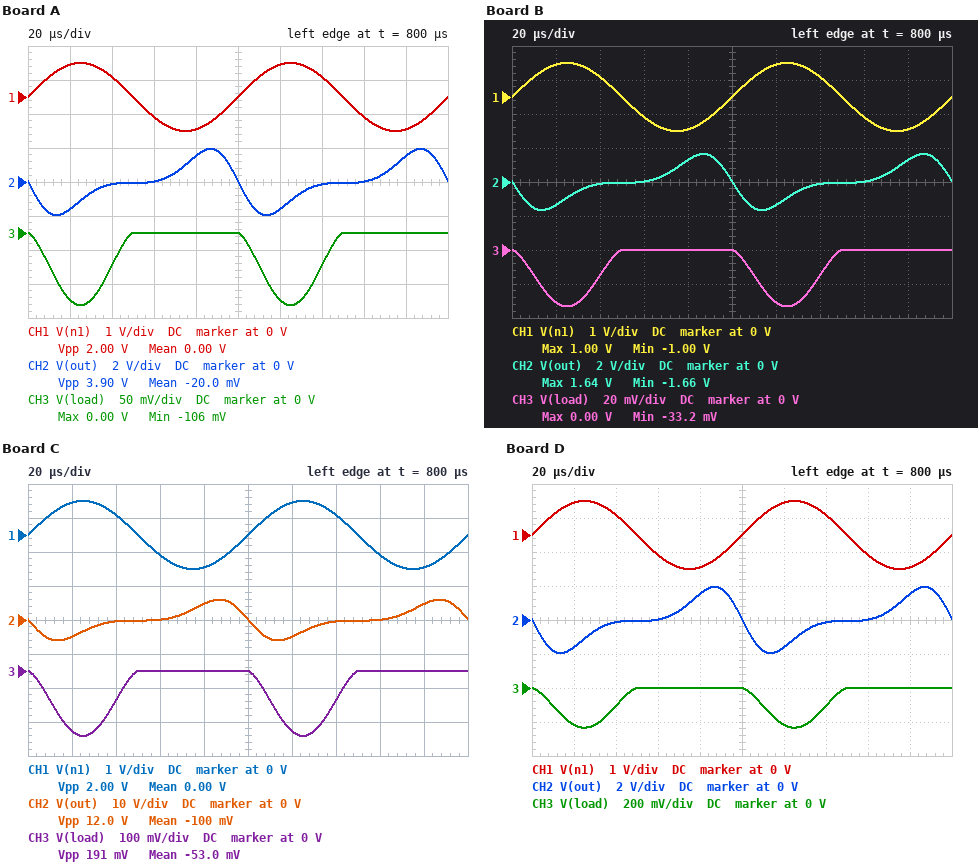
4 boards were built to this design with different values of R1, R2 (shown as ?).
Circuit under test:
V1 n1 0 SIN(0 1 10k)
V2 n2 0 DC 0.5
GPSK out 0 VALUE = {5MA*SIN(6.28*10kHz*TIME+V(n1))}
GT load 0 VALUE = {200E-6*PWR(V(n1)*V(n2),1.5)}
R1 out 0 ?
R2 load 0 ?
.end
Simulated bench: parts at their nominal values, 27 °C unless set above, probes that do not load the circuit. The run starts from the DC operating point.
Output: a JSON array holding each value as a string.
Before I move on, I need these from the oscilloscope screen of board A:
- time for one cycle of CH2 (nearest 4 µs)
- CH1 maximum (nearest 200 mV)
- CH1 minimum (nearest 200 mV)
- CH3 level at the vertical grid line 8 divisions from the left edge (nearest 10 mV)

["100 µs", "1.0 V", "-1.0 V", "0 V"]
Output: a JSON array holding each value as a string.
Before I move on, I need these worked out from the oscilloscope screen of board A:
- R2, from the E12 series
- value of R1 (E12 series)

["1.5 kΩ", "390 Ω"]
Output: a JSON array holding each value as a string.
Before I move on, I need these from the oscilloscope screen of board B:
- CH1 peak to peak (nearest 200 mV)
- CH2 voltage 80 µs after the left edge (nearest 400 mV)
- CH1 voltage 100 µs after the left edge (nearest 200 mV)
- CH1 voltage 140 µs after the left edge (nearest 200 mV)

["2.0 V", "1.2 V", "0 V", "600 mV"]
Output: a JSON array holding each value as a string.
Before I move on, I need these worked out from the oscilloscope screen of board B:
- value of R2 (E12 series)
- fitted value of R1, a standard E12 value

["470 Ω", "330 Ω"]
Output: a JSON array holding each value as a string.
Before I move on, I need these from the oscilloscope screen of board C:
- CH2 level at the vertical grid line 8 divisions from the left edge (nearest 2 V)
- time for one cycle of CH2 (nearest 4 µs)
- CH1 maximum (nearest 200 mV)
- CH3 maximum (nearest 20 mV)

["0 V", "100 µs", "1.0 V", "0 V"]
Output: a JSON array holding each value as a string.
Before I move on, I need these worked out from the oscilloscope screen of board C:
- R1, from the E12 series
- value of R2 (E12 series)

["1.2 kΩ", "2.7 kΩ"]
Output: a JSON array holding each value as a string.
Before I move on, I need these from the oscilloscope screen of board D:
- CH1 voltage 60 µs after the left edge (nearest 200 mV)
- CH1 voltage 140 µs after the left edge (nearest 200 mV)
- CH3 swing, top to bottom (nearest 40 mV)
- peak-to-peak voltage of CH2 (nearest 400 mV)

["-600 mV", "600 mV", "240 mV", "4.0 V"]
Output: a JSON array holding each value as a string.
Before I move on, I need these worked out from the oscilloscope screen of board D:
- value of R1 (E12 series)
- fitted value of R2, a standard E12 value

["390 Ω", "3.3 kΩ"]
